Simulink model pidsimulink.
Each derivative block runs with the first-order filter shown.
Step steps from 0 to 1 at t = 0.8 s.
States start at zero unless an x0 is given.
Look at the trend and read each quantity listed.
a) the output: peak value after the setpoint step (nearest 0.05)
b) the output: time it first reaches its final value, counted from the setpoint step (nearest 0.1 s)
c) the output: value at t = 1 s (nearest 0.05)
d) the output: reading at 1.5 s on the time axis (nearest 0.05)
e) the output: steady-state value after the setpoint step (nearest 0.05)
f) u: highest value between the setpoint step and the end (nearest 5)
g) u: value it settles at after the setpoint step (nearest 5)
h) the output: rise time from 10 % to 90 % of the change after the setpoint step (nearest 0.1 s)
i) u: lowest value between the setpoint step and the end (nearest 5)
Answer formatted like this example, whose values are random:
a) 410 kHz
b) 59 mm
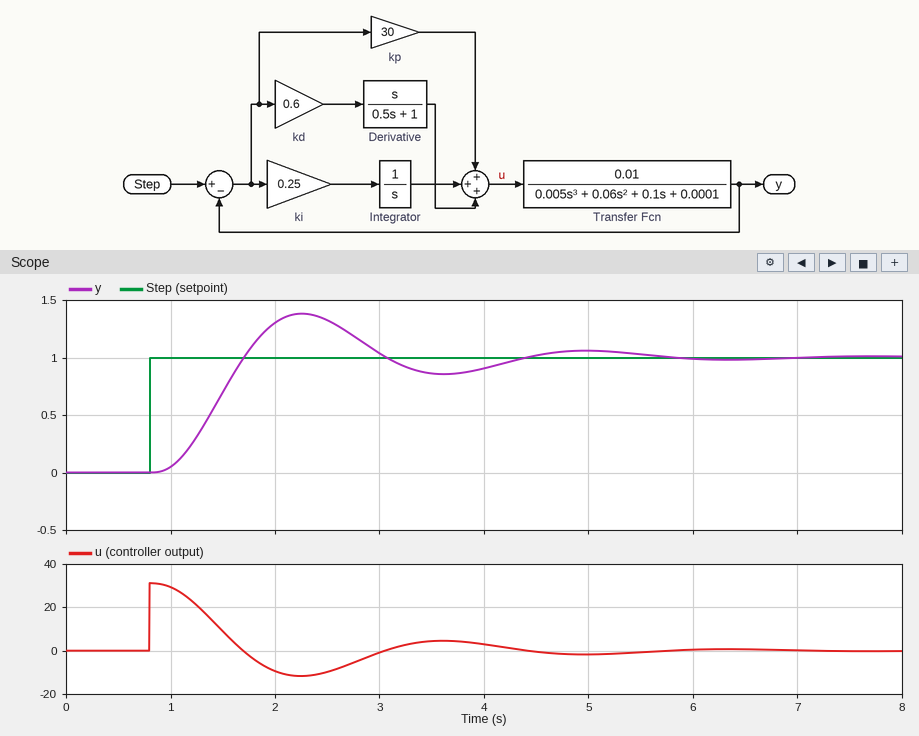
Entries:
a) 1.40
b) 0.9 s
c) 0.05
d) 0.70
e) 1.00
f) 30
g) 0
h) 0.6 s
i) -10
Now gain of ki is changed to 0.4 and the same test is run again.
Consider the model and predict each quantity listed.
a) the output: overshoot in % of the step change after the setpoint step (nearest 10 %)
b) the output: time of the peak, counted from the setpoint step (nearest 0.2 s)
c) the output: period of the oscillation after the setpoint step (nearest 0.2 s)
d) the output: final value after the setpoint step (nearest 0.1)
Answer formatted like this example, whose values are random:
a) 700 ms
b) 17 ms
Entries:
a) 40 %
b) 1.4 s
c) 2.8 s
d) 1.0
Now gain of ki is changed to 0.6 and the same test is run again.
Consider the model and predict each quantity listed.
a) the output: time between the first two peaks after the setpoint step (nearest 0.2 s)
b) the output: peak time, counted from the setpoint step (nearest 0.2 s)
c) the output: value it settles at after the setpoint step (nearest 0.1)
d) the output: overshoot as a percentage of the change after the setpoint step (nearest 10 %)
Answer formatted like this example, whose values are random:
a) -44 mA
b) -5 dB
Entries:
a) 2.8 s
b) 1.4 s
c) 1.0
d) 40 %
